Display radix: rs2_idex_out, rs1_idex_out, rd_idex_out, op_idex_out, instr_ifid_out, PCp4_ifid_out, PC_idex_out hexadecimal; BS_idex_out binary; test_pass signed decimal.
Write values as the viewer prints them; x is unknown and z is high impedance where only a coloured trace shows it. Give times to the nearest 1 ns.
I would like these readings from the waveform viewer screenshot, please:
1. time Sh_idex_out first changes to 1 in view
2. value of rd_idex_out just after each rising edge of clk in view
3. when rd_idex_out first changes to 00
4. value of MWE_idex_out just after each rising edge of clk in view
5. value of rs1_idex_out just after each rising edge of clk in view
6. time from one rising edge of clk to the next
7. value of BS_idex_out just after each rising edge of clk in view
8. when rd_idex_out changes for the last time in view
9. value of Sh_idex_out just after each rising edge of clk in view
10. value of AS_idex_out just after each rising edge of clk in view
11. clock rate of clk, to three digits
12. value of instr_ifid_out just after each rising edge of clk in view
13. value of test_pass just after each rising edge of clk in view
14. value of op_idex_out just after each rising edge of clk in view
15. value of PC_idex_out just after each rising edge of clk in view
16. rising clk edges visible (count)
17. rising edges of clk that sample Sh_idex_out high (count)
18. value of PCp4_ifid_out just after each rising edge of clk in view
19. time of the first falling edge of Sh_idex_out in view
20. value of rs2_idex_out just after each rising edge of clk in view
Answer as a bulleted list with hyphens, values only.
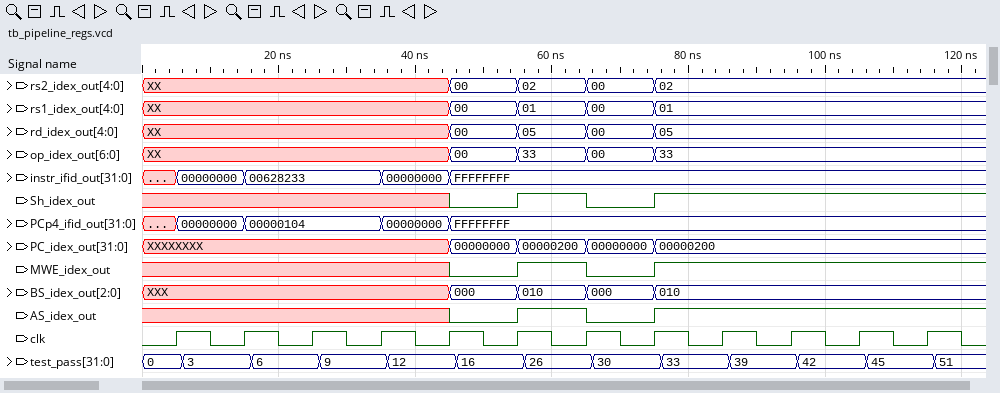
- 55 ns
- XX, XX, XX, XX, 00, 05, 00, 05, 05, 05, 05, 05
- 45 ns
- x x x x 0 1 0 1 1 1 1 1
- XX, XX, XX, XX, 00, 01, 00, 01, 01, 01, 01, 01
- 10 ns
- XXX, XXX, XXX, XXX, 000, 010, 000, 010, 010, 010, 010, 010
- 75 ns
- x x x x 0 1 0 1 1 1 1 1
- x x x x 0 1 0 1 1 1 1 1
- 100 MHz
- 00000000, 00628233, 00628233, 00000000, FFFFFFFF, FFFFFFFF, FFFFFFFF, FFFFFFFF, FFFFFFFF, FFFFFFFF, FFFFFFFF, FFFFFFFF
- 0, 3, 6, 9, 12, 16, 26, 30, 33, 39, 42, 45
- XX, XX, XX, XX, 00, 33, 00, 33, 33, 33, 33, 33
- XXXXXXXX, XXXXXXXX, XXXXXXXX, XXXXXXXX, 00000000, 00000200, 00000000, 00000200, 00000200, 00000200, 00000200, 00000200
- 12
- 5
- 00000000, 00000104, 00000104, 00000000, FFFFFFFF, FFFFFFFF, FFFFFFFF, FFFFFFFF, FFFFFFFF, FFFFFFFF, FFFFFFFF, FFFFFFFF
- 65 ns
- XX, XX, XX, XX, 00, 02, 00, 02, 02, 02, 02, 02
